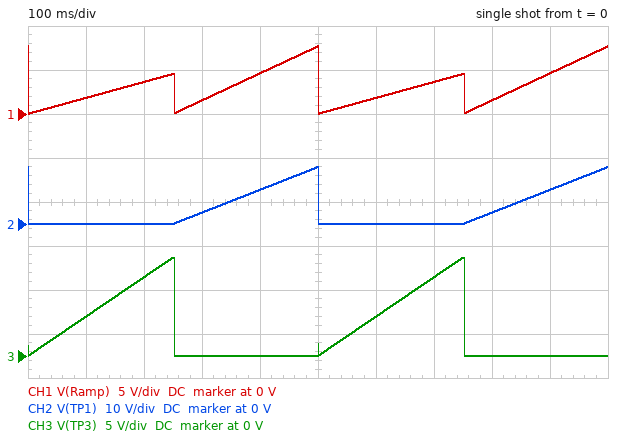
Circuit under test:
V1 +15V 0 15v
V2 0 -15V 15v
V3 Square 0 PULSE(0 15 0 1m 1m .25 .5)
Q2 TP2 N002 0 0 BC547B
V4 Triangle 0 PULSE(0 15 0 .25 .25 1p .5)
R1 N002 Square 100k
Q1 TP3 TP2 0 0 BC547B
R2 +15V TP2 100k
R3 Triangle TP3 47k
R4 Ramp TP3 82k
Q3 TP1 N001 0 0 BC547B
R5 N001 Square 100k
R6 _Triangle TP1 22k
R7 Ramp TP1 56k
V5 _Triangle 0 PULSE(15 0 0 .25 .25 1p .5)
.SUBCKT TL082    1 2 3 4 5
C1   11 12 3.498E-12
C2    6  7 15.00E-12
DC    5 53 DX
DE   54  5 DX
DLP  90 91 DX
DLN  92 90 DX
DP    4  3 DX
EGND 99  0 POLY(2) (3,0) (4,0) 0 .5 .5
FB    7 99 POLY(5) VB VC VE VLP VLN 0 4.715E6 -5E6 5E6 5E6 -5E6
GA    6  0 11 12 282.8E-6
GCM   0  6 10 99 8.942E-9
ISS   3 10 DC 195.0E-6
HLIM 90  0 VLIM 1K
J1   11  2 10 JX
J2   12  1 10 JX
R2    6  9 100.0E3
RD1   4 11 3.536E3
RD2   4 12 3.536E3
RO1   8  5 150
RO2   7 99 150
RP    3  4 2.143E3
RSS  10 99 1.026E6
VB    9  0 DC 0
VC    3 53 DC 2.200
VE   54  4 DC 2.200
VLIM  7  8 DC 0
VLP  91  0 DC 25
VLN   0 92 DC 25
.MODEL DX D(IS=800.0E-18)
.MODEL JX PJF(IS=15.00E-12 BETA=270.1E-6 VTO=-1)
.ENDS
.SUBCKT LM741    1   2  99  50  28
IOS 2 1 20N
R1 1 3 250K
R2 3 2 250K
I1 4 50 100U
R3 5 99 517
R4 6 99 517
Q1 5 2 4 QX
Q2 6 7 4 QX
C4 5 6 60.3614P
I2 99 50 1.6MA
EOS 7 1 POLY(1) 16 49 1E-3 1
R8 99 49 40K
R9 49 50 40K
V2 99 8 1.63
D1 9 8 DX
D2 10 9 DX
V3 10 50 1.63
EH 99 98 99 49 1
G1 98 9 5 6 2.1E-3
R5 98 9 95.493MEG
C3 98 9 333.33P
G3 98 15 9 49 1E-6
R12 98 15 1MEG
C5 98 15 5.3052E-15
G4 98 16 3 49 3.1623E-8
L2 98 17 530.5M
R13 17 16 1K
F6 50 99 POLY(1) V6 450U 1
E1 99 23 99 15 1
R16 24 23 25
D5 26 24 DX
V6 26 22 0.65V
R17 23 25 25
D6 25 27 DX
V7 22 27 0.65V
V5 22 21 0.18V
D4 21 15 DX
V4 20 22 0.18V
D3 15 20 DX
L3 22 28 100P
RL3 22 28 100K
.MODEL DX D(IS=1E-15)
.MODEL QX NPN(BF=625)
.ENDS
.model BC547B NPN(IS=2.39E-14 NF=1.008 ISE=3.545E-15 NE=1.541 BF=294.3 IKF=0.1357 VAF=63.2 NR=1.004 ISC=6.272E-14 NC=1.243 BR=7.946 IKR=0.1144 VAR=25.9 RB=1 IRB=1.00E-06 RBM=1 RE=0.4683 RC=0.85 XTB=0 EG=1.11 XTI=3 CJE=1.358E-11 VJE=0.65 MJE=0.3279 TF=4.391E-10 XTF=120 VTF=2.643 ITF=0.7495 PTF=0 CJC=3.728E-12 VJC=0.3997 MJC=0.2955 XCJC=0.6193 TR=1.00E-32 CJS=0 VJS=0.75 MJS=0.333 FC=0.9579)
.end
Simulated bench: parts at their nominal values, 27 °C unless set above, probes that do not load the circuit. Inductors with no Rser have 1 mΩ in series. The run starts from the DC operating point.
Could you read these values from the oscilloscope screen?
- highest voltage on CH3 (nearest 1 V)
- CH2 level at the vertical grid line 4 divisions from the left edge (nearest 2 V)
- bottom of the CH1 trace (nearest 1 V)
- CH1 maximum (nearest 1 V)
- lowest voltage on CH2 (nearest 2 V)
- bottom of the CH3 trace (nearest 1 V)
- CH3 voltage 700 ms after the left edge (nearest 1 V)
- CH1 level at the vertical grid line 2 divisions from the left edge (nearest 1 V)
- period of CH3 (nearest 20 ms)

11 V
8 V
0 V
8 V
0 V
0 V
9 V
4 V
500 ms
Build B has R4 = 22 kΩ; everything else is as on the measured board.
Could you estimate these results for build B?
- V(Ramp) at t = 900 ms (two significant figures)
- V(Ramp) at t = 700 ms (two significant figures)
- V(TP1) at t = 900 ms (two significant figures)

2.0 V
5.4 V
7.0 V
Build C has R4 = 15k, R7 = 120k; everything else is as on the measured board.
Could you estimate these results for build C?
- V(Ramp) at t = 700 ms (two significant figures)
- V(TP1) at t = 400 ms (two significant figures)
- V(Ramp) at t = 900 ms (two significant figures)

7.9 V
7.7 V
870 mV
